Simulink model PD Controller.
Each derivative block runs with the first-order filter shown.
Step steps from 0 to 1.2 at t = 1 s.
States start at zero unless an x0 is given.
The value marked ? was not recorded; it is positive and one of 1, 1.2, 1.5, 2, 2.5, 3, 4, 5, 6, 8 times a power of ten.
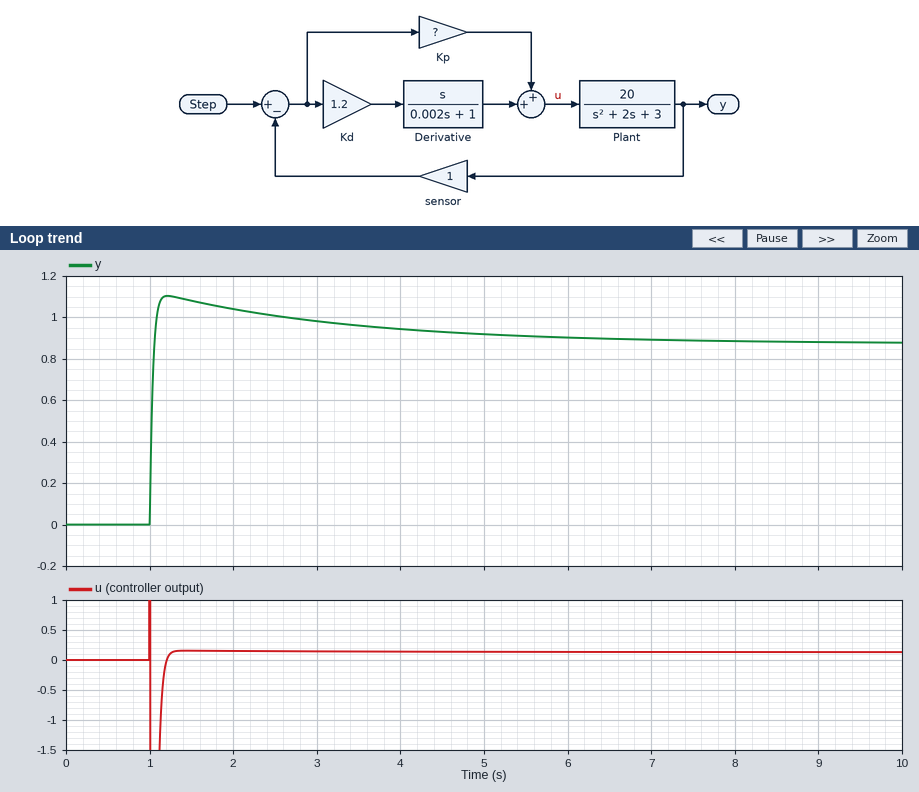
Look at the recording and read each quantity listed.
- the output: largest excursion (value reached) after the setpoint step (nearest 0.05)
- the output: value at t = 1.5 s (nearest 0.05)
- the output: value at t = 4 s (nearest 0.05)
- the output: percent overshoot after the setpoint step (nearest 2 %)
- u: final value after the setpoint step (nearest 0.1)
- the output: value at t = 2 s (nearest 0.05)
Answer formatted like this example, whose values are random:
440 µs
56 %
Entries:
1.10
1.10
0.95
26 %
0.1
1.05
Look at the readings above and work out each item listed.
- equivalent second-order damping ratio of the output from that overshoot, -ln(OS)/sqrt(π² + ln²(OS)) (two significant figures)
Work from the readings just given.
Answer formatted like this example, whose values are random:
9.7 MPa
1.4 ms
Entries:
0.39
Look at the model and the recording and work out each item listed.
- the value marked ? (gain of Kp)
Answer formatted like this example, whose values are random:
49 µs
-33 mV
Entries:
0.4
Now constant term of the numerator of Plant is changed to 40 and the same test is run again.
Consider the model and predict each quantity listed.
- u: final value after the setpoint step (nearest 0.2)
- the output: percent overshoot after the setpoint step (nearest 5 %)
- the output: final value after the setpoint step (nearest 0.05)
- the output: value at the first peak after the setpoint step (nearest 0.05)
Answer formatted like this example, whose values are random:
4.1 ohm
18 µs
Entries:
0.0
15 %
1.00
1.15
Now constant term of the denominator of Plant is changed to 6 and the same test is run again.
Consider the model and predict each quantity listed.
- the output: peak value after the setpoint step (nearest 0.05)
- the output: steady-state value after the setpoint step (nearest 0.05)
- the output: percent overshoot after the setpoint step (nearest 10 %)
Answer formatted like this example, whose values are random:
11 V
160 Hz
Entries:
1.10
0.70
60 %
